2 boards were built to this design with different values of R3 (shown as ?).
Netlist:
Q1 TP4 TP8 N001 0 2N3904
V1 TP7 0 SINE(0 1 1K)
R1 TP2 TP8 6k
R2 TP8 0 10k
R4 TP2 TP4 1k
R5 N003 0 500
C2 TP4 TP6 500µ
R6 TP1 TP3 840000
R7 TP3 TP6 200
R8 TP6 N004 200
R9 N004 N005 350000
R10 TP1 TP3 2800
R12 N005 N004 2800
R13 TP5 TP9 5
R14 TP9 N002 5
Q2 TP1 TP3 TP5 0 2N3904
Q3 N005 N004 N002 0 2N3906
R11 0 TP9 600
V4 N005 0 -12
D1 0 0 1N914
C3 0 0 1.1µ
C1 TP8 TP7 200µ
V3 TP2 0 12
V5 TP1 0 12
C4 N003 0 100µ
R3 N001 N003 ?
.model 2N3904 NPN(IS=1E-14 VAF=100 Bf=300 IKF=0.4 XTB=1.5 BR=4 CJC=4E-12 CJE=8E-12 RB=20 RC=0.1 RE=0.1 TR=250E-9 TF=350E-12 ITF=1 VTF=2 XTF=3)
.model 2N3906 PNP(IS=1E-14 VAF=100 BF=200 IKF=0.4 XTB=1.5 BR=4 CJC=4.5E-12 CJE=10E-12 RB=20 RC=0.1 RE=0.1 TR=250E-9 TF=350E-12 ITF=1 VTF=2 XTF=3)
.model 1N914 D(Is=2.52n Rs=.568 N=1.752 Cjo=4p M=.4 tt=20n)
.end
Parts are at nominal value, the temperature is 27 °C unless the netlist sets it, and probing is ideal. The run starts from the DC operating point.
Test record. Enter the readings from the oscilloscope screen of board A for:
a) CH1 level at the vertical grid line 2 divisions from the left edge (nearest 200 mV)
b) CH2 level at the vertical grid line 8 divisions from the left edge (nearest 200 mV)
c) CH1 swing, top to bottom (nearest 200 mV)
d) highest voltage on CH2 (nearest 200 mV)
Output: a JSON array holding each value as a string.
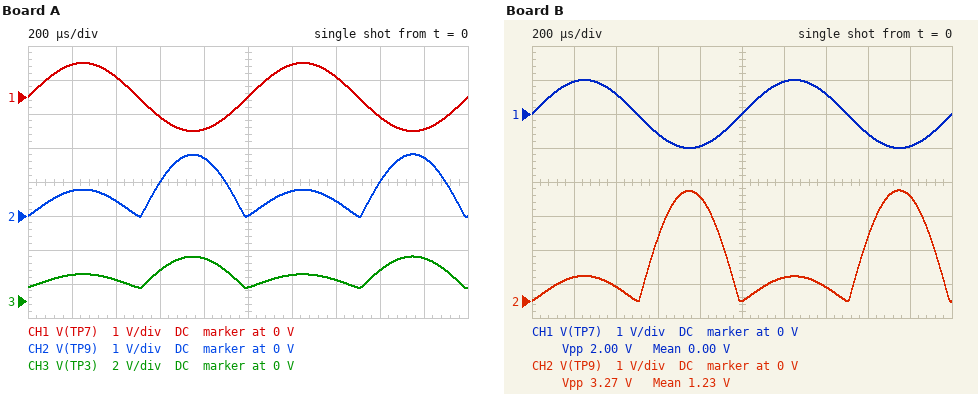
["600 mV", "1.0 V", "2.0 V", "1.8 V"]
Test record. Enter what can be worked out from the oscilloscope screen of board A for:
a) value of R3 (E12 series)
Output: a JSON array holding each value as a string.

["270 Ω"]
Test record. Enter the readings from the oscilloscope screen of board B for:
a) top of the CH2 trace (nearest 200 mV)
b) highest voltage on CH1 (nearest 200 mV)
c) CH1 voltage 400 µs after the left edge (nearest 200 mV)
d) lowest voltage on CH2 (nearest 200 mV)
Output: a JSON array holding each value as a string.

["3.2 V", "1.0 V", "600 mV", "0 V"]
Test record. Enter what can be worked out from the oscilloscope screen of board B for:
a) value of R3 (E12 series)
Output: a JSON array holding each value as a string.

["150 Ω"]
